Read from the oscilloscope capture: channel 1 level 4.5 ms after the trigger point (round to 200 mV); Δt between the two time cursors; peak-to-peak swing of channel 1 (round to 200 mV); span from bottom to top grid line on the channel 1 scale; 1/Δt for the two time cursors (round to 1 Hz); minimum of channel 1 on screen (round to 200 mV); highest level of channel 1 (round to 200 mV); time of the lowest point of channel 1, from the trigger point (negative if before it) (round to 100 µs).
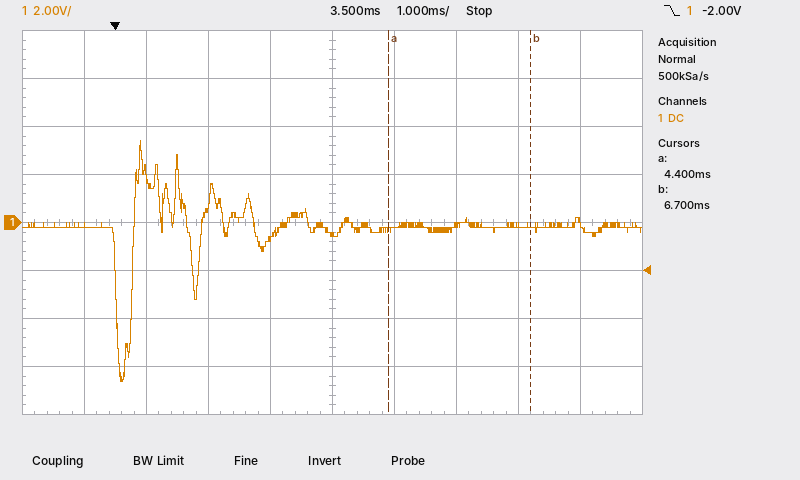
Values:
-200 mV
2.3 ms
10.0 V
16 V
435 Hz
-6.6 V
3.4 V
+100 µs
